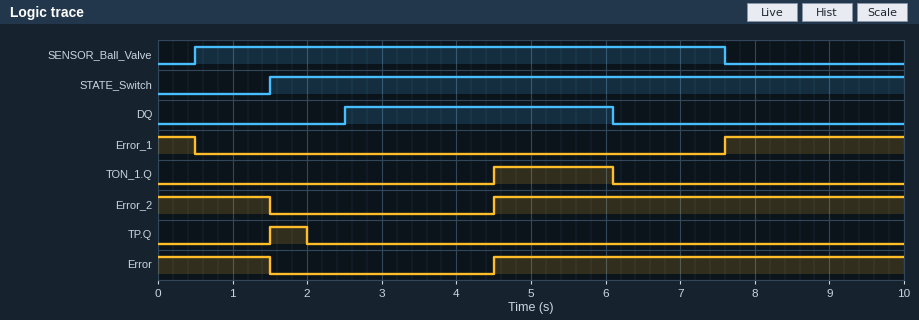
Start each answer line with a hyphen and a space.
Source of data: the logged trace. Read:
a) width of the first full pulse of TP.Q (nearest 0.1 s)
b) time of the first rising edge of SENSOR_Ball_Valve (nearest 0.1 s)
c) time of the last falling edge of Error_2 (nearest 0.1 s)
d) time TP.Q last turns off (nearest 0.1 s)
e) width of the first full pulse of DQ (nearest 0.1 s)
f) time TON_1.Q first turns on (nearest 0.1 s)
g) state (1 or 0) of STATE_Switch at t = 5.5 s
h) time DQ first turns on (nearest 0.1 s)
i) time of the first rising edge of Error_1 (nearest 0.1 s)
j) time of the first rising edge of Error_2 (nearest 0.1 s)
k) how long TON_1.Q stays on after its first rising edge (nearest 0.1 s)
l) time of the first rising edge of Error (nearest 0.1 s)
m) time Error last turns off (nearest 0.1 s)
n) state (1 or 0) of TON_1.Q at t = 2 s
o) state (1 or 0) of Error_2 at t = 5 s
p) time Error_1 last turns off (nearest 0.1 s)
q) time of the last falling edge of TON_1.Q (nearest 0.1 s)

- 0.5 s
- 0.5 s
- 1.5 s
- 2.0 s
- 3.6 s
- 4.5 s
- 1
- 2.5 s
- 7.6 s
- 4.5 s
- 1.6 s
- 4.5 s
- 1.5 s
- 0
- 1
- 0.5 s
- 6.1 s
